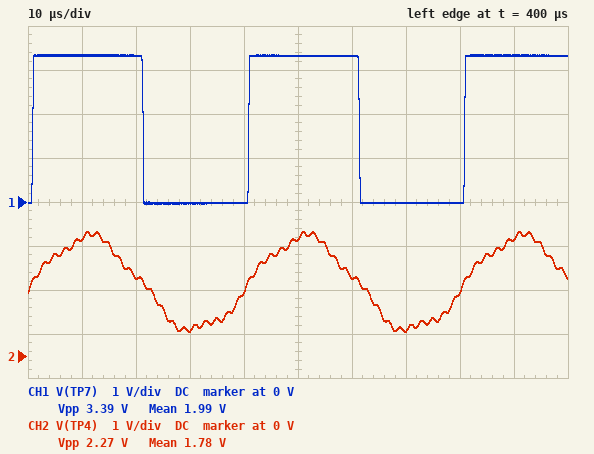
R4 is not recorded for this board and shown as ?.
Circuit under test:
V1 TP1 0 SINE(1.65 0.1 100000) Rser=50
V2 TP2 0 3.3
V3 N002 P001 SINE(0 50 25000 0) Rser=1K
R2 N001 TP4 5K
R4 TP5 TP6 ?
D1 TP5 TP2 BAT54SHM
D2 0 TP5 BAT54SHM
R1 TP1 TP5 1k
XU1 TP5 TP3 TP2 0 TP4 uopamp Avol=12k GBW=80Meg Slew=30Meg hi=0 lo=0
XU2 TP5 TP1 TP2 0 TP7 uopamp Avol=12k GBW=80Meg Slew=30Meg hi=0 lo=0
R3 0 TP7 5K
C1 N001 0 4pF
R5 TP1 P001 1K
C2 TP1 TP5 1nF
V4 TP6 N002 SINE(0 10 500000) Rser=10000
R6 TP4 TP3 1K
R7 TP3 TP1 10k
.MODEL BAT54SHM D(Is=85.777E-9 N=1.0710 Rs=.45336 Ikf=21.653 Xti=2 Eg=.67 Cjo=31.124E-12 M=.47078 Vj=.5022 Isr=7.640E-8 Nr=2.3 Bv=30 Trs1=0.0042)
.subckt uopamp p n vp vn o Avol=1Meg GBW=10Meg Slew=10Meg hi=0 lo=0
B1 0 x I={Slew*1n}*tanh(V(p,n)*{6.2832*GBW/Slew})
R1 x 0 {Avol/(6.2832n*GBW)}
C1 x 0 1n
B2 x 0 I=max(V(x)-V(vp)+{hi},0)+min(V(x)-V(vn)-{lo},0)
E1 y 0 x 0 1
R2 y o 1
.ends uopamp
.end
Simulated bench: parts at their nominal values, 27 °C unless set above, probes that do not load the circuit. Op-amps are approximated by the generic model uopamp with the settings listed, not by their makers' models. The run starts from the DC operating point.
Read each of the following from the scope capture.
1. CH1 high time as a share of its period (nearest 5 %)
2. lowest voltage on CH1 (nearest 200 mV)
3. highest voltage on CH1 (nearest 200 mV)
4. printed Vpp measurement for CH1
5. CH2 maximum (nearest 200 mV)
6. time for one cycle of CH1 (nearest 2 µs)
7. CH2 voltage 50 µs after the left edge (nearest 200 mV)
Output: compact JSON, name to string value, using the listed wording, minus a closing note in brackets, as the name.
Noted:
{"CH1 high time as a share of its period": "50 %", "lowest voltage on CH1": "0 V", "highest voltage on CH1": "3.4 V", "printed Vpp measurement for CH1": "3.39 V", "CH2 maximum": "2.8 V", "time for one cycle of CH1": "40 µs", "CH2 voltage 50 µs after the left edge": "2.6 V"}
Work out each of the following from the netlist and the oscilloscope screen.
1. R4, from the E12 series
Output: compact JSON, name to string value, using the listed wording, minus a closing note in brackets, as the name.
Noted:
{"R4, from the E12 series": "39 kΩ"}
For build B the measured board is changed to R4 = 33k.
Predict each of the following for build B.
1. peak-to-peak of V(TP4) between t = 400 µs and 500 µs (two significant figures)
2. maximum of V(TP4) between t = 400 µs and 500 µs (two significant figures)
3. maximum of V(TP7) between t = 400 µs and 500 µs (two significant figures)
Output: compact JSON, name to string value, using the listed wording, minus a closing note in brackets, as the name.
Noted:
{"peak-to-peak of V(TP4) between t = 400 µs and 500 µs": "2.6 V", "maximum of V(TP4) between t = 400 µs and 500 µs": "3.0 V", "maximum of V(TP7) between t = 400 µs and 500 µs": "3.3 V"}
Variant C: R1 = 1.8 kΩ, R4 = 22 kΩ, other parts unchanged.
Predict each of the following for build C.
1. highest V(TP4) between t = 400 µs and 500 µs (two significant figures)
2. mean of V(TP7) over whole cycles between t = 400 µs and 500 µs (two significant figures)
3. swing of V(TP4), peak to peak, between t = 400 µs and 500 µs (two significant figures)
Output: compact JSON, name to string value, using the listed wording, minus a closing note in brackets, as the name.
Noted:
{"highest V(TP4) between t = 400 µs and 500 µs": "3.3 V", "mean of V(TP7) over whole cycles between t = 400 µs and 500 µs": "1.6 V", "swing of V(TP4), peak to peak, between t = 400 µs and 500 µs": "3.4 V"}
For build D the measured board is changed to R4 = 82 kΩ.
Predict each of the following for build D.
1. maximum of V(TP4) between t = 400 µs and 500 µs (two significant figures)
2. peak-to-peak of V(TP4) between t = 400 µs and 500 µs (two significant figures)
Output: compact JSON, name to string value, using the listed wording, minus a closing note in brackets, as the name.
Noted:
{"maximum of V(TP4) between t = 400 µs and 500 µs": "2.3 V", "peak-to-peak of V(TP4) between t = 400 µs and 500 µs": "1.3 V"}
